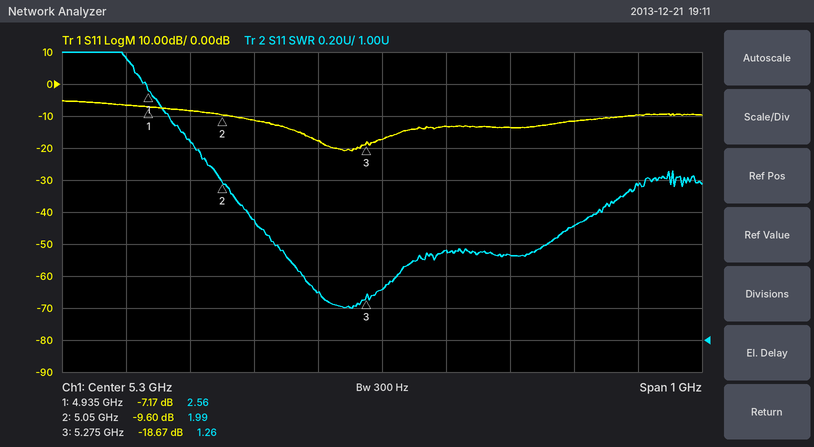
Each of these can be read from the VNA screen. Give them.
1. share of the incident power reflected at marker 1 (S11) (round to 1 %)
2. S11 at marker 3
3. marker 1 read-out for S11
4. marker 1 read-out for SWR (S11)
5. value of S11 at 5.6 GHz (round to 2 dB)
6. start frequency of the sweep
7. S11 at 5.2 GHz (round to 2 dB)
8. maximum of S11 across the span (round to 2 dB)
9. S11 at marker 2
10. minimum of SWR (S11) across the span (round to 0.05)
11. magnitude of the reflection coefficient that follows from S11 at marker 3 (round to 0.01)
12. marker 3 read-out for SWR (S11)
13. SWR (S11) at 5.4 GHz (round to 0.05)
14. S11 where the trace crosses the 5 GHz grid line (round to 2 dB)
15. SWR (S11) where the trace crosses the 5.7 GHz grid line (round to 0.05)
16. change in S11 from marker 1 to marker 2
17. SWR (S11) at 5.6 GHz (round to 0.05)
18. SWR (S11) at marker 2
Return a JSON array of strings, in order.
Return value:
["19 %", "-18.67 dB", "-7.17 dB", "2.56", "-12 dB", "4.8 GHz", "-18 dB", "-6 dB", "-9.60 dB", "1.20", "0.12", "1.26", "1.55", "-8 dB", "1.95", "-2.43 dB", "1.70", "1.99"]
